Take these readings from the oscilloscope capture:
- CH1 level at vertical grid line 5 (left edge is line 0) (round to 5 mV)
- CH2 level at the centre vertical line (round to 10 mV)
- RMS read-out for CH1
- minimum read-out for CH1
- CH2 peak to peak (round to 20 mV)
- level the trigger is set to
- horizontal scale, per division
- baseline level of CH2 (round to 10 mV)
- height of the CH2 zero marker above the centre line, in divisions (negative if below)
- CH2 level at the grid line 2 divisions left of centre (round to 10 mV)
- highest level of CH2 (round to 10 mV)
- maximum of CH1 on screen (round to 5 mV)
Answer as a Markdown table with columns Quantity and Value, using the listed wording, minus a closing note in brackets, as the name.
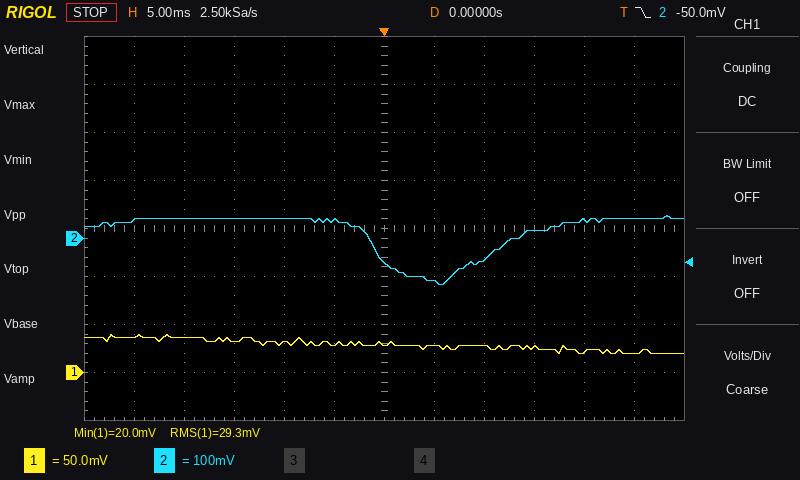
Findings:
| Quantity | Value |
|---|---|
| CH1 level at vertical grid line 5 (left edge is line 0) | 30 mV |
| CH2 level at the centre vertical line | -50 mV |
| RMS read-out for CH1 | 29.3 mV |
| minimum read-out for CH1 | 20.0 mV |
| CH2 peak to peak | 140 mV |
| level the trigger is set to | -50.0 mV |
| horizontal scale, per division | 5 ms |
| baseline level of CH2 | 40 mV |
| height of the CH2 zero marker above the centre line, in divisions | -0.2 div |
| CH2 level at the grid line 2 divisions left of centre | 40 mV |
| highest level of CH2 | 50 mV |
| maximum of CH1 on screen | 40 mV |
